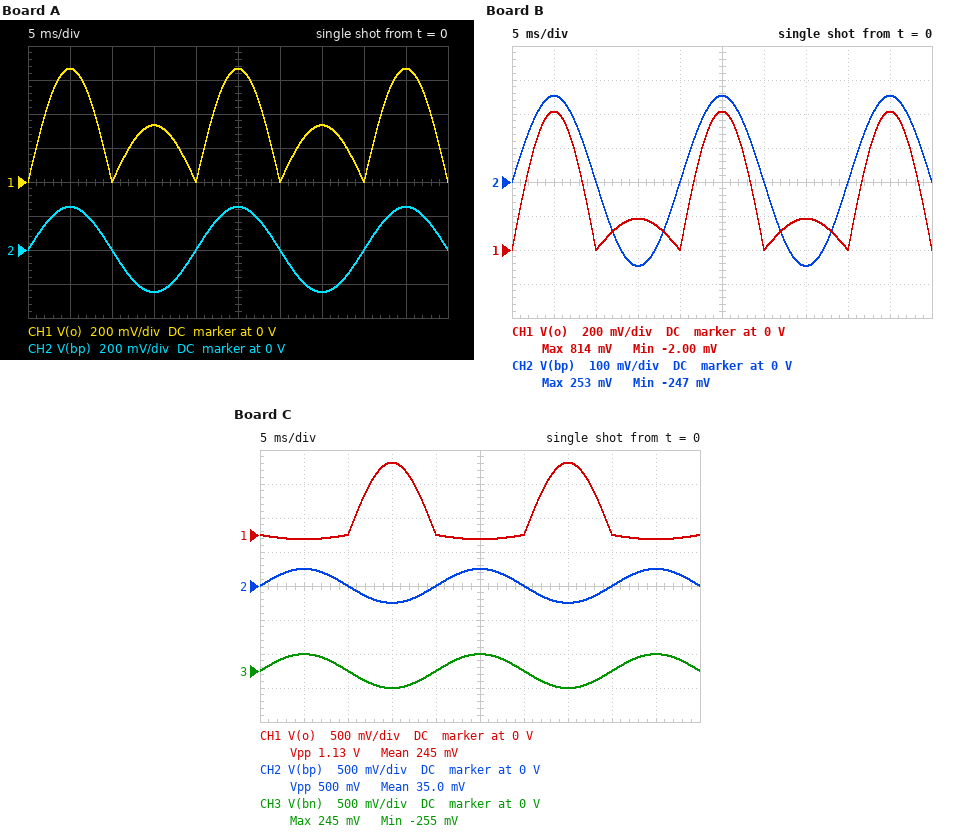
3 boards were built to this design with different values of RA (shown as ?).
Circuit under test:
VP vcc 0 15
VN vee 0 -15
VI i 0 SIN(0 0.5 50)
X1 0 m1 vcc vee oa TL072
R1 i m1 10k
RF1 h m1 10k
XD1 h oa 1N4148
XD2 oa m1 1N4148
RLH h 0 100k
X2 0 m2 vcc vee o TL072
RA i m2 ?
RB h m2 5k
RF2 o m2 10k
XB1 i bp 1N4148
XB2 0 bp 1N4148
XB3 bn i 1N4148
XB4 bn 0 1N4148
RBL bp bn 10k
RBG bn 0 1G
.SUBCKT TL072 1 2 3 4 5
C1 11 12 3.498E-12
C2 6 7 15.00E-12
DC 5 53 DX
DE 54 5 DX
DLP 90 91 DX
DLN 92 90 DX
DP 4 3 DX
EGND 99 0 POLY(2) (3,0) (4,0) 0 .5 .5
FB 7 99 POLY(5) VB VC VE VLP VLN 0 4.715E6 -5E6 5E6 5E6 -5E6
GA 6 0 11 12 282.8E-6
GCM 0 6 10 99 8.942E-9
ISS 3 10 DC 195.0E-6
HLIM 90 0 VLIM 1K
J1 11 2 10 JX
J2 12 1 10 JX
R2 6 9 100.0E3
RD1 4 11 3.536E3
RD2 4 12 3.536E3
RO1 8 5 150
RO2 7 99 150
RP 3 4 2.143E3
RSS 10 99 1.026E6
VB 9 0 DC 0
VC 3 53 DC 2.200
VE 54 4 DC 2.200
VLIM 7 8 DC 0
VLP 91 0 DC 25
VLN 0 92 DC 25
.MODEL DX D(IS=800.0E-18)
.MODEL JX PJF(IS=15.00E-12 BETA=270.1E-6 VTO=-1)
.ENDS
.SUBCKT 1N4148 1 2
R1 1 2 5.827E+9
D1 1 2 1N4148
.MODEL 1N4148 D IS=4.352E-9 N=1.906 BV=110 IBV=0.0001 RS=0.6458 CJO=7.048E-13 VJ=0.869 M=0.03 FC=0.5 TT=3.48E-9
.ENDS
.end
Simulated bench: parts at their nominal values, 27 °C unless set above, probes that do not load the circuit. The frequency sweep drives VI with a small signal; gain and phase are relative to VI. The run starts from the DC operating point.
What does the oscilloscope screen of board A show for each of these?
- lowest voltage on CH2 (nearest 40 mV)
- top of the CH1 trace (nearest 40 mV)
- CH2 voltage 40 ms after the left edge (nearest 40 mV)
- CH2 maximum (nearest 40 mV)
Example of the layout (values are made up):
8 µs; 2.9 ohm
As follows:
-240 mV; 680 mV; 0 V; 240 mV
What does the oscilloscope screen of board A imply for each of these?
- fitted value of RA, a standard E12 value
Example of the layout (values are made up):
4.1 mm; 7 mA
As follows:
15 kΩ
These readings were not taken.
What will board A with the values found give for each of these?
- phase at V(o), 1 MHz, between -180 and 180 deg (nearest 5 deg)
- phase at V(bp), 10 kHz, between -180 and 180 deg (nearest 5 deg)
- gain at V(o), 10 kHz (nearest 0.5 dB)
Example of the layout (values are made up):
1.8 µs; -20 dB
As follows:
145 deg; 0 deg; -0.5 dB
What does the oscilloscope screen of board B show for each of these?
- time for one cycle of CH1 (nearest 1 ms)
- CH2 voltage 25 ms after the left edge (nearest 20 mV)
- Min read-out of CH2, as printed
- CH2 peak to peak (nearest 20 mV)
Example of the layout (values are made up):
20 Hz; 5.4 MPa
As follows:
20 ms; 260 mV; -247 mV; 500 mV
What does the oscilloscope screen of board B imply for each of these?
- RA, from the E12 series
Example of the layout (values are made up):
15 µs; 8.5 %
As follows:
27 kΩ
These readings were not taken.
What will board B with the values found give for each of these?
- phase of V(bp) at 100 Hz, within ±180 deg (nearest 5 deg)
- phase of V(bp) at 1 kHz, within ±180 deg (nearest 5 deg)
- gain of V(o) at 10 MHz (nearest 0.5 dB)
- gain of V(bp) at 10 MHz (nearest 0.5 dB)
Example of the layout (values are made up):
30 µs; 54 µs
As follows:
0 deg; 0 deg; -22.0 dB; -6.0 dB
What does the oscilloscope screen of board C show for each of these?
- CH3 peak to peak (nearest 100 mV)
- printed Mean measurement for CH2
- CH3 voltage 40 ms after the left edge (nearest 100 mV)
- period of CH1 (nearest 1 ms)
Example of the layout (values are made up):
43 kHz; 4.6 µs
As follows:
500 mV; 35.0 mV; 0 V; 20 ms
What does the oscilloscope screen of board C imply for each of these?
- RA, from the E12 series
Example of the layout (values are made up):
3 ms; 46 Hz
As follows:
4.7 kΩ
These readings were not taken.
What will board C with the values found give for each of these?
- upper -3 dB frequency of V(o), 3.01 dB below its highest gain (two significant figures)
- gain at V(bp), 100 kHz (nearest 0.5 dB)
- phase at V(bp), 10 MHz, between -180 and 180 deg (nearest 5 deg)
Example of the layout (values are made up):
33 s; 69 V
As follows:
1.1 MHz; -6.0 dB; 0 deg
